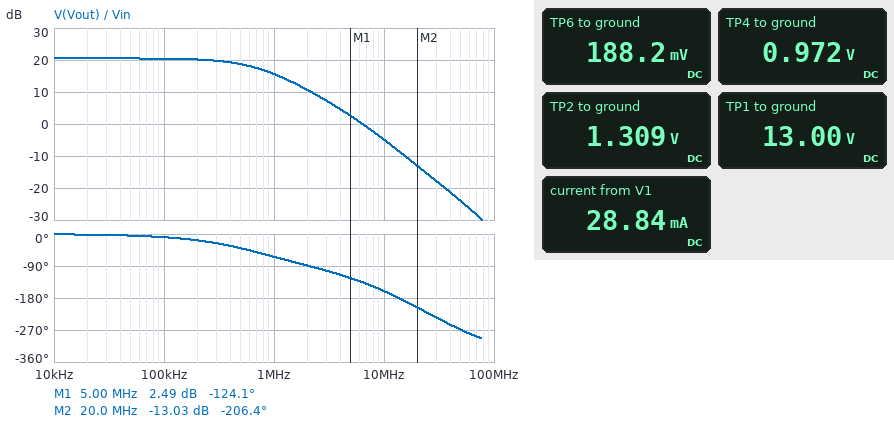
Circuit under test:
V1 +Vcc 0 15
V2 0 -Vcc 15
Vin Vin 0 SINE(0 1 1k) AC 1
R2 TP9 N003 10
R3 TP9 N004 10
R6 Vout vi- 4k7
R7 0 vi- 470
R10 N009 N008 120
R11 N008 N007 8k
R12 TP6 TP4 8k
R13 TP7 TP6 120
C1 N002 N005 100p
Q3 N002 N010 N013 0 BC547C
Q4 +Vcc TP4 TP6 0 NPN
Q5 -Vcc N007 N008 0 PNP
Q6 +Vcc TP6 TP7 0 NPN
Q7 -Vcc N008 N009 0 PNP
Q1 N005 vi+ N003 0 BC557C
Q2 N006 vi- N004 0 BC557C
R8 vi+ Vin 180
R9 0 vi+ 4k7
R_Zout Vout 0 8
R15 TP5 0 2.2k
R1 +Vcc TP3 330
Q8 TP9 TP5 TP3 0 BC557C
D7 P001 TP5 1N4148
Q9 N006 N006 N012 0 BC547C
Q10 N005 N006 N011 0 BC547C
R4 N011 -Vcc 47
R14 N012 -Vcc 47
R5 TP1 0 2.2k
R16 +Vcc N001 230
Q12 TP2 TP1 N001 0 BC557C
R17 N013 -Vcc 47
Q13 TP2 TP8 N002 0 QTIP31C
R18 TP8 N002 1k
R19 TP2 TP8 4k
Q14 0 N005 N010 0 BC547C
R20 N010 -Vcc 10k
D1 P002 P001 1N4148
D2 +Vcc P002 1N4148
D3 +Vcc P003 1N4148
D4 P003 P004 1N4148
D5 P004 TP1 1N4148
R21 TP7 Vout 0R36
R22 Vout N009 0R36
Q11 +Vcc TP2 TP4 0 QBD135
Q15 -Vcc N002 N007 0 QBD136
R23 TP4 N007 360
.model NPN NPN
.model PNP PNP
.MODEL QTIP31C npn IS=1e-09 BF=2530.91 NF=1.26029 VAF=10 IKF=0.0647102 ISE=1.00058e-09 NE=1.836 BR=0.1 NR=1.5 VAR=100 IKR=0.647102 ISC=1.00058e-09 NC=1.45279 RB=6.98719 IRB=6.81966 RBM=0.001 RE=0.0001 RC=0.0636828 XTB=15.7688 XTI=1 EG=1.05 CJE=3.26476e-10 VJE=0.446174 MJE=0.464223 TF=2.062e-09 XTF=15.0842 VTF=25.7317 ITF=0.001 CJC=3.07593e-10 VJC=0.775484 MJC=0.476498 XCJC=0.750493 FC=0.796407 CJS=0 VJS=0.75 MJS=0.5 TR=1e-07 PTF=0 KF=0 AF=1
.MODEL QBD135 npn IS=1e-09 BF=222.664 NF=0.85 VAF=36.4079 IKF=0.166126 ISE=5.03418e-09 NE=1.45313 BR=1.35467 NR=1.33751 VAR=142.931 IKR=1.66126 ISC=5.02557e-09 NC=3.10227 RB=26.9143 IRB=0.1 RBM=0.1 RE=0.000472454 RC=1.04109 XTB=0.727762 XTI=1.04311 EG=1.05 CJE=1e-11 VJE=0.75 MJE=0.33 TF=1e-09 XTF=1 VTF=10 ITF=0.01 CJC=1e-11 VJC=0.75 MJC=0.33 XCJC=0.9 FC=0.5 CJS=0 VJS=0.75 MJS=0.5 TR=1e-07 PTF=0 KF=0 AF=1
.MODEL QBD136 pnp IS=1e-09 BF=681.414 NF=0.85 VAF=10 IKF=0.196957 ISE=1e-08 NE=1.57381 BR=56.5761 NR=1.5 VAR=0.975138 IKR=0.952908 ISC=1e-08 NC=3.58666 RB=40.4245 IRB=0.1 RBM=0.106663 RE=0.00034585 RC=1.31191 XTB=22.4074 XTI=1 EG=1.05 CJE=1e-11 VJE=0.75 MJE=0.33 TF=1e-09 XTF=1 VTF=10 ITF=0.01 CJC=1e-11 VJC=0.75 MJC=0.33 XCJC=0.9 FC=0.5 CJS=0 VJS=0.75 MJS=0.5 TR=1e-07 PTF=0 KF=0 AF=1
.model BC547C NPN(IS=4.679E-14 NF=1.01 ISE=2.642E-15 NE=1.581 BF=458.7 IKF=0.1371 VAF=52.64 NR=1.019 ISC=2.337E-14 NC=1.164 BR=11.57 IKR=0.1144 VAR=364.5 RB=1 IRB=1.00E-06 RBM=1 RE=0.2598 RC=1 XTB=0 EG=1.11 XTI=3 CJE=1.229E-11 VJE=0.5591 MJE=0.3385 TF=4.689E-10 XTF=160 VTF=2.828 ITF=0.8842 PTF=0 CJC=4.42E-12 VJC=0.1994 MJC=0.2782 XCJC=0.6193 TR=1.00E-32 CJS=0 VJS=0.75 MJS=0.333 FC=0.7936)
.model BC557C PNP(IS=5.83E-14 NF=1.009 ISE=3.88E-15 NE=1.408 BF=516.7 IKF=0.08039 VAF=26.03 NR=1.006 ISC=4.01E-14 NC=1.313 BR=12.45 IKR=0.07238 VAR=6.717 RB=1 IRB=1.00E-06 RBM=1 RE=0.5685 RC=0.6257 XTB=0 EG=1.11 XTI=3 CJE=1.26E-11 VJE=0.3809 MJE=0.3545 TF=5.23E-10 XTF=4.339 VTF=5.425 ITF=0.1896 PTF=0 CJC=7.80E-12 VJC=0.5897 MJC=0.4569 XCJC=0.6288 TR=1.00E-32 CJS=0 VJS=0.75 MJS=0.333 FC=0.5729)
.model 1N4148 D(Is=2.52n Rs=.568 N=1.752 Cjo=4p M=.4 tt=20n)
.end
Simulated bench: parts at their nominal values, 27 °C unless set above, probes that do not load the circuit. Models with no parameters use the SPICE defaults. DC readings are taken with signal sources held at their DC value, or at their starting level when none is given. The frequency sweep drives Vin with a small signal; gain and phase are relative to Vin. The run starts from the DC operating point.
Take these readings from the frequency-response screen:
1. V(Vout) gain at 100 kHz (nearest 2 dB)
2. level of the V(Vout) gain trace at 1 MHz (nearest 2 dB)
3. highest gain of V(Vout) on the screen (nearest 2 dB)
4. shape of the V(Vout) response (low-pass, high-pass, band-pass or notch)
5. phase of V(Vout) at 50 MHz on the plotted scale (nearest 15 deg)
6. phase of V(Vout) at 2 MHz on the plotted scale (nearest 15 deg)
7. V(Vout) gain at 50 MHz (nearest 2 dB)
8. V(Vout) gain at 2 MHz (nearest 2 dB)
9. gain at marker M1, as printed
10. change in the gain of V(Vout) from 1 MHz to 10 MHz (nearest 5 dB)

20 dB
16 dB
20 dB
low-pass
-270 deg
-90 deg
-24 dB
10 dB
2.49 dB
-20 dB
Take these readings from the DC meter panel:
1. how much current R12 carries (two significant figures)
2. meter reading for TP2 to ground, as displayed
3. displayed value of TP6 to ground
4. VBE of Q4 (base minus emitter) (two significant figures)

98 µA
1.309 V
188.2 mV
780 mV
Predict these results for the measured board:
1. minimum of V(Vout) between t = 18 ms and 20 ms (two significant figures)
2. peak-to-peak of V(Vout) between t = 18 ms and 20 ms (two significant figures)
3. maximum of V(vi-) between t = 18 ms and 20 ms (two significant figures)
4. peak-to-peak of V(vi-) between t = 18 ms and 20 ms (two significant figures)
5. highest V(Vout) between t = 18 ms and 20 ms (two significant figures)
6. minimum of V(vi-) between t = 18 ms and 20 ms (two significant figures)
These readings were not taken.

-11 V
21 V
960 mV
1.9 V
11 V
-960 mV
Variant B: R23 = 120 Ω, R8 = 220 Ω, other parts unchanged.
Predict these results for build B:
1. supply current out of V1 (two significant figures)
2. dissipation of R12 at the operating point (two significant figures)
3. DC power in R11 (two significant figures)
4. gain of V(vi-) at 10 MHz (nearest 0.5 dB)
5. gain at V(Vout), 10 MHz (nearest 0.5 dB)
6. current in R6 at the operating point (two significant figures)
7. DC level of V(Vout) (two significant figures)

39 mA
76 µW
77 µW
-8.5 dB
-5.5 dB
550 nA
-1.5 mV
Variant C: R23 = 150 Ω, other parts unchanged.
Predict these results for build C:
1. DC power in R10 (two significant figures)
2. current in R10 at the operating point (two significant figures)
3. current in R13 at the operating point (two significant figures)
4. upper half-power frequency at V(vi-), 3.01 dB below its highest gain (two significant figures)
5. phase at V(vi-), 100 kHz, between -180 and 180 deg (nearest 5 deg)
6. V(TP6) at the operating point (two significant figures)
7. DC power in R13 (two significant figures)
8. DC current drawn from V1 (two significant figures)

370 µW
1.8 mA
1.4 mA
630 kHz
-10 deg
170 mV
240 µW
36 mA
